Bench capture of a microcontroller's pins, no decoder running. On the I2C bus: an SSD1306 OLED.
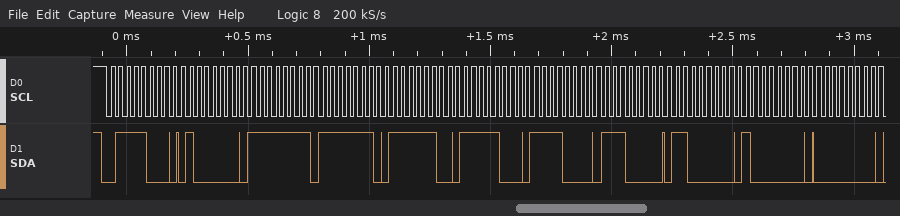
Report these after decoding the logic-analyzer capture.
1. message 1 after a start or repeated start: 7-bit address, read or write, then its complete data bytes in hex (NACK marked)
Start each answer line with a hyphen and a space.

- 0x3C write: 40 FF FE FC F8 F0 E0 C0 80 00
